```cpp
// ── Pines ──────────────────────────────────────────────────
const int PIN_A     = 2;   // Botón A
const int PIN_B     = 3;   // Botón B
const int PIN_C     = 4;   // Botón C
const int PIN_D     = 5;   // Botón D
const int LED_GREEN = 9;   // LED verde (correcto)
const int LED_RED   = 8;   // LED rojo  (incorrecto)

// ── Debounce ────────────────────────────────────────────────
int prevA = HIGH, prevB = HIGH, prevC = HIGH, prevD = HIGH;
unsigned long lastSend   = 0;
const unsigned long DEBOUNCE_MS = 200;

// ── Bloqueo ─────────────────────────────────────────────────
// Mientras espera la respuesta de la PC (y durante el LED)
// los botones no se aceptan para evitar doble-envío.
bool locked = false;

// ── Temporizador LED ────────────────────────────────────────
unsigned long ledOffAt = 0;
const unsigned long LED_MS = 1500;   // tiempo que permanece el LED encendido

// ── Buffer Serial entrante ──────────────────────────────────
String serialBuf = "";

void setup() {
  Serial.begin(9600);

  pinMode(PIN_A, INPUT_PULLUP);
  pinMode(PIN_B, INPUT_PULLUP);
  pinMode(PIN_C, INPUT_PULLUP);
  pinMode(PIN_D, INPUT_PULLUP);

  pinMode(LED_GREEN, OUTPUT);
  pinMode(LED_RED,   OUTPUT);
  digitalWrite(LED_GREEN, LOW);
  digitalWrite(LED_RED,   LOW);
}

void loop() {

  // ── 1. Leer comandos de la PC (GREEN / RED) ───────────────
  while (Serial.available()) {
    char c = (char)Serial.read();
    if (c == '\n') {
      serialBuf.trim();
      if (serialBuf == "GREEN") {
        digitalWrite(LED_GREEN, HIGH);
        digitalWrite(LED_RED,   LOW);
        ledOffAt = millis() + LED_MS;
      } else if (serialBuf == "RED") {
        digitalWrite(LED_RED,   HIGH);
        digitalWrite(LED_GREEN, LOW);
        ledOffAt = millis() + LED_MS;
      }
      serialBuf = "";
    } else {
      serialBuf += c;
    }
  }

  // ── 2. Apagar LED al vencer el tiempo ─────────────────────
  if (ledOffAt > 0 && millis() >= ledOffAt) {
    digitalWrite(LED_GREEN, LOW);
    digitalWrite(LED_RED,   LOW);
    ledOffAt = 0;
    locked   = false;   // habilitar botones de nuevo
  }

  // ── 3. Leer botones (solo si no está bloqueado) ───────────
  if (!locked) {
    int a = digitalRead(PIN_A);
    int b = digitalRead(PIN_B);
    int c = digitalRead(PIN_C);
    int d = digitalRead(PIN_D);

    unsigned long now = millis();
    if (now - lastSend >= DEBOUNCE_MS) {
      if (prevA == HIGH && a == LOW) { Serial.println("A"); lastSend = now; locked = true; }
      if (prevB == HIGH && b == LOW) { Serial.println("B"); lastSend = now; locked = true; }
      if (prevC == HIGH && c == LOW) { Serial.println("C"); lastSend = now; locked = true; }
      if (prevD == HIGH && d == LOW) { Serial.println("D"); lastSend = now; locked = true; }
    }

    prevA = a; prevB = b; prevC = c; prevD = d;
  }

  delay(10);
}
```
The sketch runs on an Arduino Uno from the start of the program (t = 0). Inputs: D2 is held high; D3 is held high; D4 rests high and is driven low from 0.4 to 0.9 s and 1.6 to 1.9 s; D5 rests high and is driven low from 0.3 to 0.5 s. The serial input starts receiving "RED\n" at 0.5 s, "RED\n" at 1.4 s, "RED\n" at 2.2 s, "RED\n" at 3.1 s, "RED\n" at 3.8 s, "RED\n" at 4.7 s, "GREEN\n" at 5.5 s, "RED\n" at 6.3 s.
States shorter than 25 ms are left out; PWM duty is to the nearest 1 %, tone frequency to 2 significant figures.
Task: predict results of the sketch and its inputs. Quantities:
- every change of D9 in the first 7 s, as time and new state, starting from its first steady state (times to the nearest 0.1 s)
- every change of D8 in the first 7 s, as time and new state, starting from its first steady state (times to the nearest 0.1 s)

0 s low; 5.5 s high; 6.3 s low
0 s low; 0.5 s high; 5.5 s low; 6.3 s high
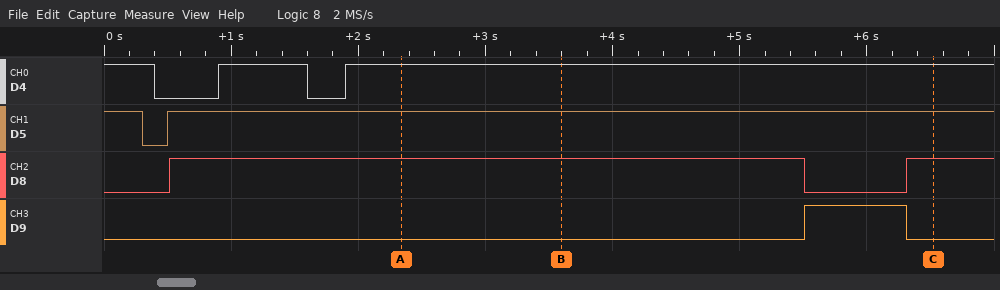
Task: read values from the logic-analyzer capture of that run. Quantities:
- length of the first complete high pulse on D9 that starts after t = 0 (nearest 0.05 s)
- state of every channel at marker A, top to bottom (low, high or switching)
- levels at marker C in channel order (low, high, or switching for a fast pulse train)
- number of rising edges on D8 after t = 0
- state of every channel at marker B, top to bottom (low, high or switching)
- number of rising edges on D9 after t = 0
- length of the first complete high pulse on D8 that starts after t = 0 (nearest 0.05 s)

0.80 s
D4 high, D5 high, D8 high, D9 low
D4 high, D5 high, D8 high, D9 low
2
D4 high, D5 high, D8 high, D9 low
1
5.00 s
